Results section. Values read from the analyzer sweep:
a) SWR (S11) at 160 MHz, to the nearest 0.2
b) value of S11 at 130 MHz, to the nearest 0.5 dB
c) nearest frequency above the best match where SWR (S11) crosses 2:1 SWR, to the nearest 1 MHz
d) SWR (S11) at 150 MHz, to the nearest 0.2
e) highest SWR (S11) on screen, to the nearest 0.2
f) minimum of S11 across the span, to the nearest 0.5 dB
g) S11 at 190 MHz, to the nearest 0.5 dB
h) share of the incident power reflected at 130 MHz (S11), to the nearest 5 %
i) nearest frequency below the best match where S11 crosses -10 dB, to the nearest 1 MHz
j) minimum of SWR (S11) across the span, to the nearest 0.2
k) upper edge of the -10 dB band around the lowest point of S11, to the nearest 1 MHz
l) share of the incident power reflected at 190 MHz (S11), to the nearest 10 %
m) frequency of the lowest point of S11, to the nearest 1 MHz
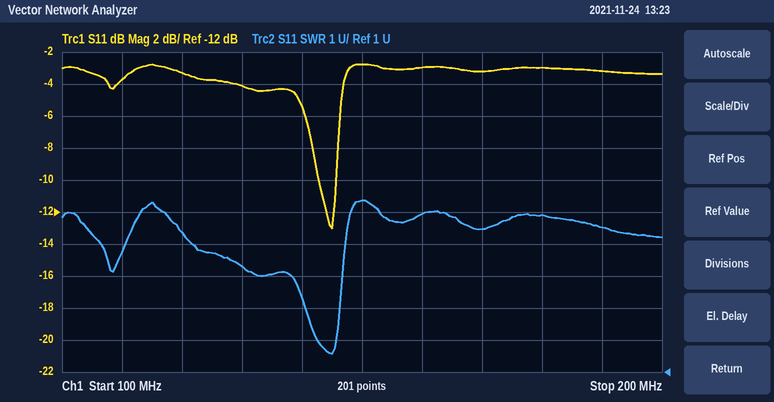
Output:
6.0
-4.0 dB
146 MHz
6.4
6.4
-13.0 dB
-3.0 dB
40 %
143 MHz
1.6
146 MHz
50 %
145 MHz
